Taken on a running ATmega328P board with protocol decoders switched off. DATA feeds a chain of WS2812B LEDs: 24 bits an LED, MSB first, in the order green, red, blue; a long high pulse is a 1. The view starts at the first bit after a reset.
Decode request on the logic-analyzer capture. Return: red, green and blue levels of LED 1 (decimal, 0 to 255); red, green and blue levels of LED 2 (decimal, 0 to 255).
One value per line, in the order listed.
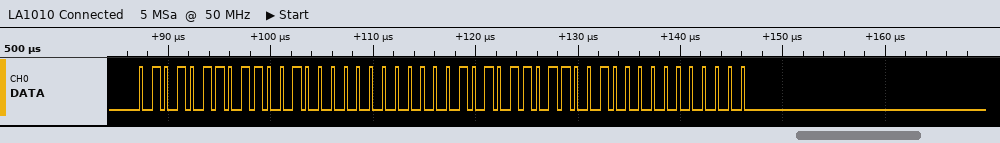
200, 86, 0
200, 86, 0
